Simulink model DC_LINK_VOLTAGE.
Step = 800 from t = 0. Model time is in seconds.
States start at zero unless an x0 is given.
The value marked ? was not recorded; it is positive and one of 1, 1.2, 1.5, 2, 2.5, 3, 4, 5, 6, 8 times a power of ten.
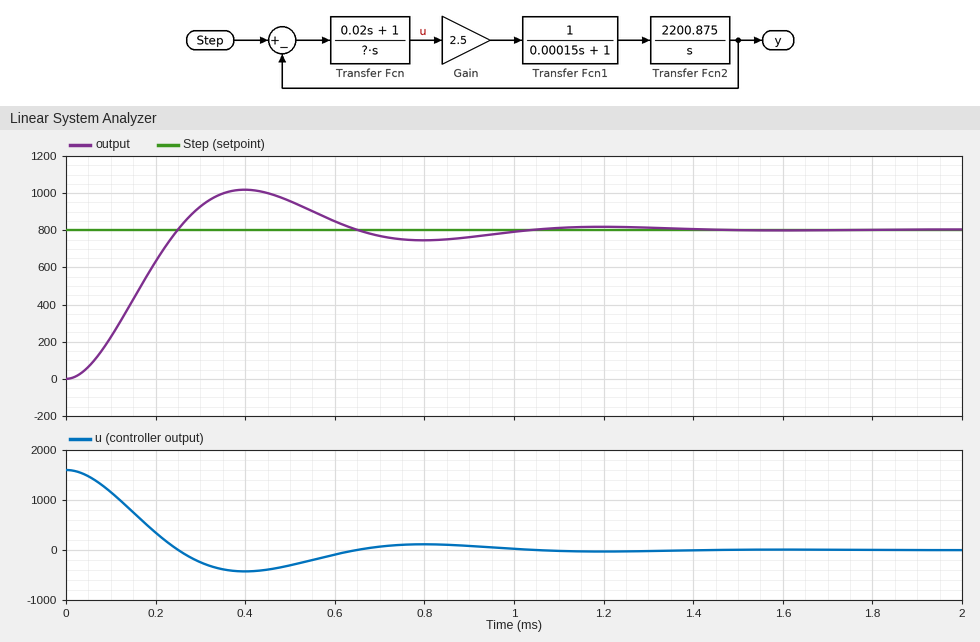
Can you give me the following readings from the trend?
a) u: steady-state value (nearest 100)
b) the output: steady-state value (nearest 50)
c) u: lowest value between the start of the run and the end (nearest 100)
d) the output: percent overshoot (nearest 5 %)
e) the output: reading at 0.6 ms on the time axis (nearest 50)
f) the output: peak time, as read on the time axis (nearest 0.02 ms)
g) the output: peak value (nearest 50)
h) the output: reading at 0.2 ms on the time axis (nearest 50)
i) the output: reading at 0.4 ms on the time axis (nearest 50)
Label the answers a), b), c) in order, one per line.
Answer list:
a) 0
b) 800
c) -400
d) 25 %
e) 850
f) 0.40 ms
g) 1000
h) 650
i) 1000
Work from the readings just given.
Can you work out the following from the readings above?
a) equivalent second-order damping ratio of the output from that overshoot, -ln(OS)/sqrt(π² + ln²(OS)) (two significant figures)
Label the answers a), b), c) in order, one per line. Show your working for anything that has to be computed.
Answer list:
a) ln(0.25) = -1.386; 1.386 / sqrt(9.870 + 1.922) = 0.40
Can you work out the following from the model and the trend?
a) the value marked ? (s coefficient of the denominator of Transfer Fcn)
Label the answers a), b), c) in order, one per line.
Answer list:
a) 0.01
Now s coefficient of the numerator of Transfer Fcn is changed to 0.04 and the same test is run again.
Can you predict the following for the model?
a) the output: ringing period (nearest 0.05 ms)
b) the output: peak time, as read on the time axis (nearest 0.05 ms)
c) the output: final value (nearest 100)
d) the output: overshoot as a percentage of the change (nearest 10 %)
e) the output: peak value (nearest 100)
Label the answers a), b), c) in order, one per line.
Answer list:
a) 0.55 ms
b) 0.25 ms
c) 800
d) 40 %
e) 1100
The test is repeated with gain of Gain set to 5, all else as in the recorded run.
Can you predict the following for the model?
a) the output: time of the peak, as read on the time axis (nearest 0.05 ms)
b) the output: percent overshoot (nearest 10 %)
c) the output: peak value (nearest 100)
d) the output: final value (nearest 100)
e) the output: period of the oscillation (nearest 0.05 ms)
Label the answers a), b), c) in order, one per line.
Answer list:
a) 0.25 ms
b) 40 %
c) 1100
d) 800
e) 0.55 ms
